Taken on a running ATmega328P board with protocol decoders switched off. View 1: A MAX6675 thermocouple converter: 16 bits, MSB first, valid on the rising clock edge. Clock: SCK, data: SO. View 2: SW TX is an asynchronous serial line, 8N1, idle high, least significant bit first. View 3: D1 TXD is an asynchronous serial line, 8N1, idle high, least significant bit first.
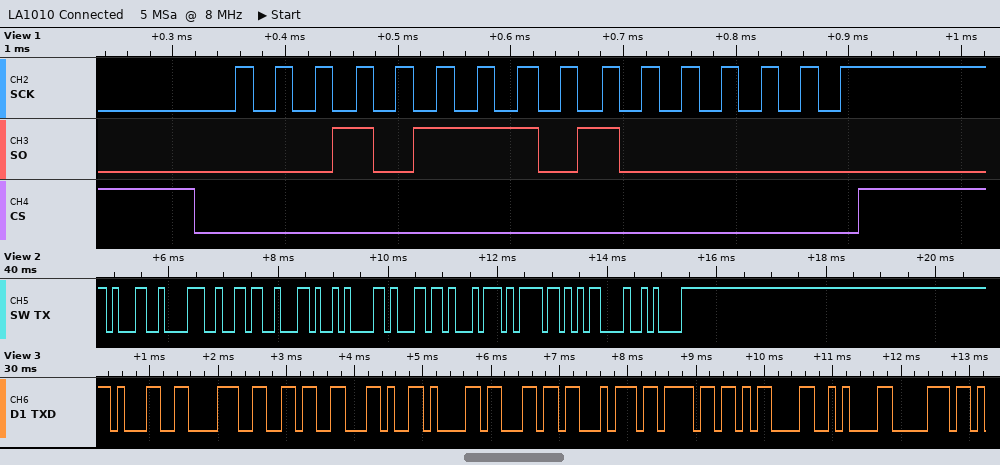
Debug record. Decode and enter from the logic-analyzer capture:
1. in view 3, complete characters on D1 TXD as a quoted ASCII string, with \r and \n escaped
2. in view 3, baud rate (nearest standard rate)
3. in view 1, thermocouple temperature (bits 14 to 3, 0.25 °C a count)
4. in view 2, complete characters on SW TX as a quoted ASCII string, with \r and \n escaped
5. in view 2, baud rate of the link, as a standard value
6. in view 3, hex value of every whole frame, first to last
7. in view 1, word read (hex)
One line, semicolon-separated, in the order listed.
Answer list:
"186,alto\r\np"; 9600 baud; 186.00 °C; "186,alto\r\n"; 9600 baud; 0x31 0x38 0x36 0x2C 0x61 0x6C 0x74 0x6F 0x0D 0x0A 0x70; 0x1740
